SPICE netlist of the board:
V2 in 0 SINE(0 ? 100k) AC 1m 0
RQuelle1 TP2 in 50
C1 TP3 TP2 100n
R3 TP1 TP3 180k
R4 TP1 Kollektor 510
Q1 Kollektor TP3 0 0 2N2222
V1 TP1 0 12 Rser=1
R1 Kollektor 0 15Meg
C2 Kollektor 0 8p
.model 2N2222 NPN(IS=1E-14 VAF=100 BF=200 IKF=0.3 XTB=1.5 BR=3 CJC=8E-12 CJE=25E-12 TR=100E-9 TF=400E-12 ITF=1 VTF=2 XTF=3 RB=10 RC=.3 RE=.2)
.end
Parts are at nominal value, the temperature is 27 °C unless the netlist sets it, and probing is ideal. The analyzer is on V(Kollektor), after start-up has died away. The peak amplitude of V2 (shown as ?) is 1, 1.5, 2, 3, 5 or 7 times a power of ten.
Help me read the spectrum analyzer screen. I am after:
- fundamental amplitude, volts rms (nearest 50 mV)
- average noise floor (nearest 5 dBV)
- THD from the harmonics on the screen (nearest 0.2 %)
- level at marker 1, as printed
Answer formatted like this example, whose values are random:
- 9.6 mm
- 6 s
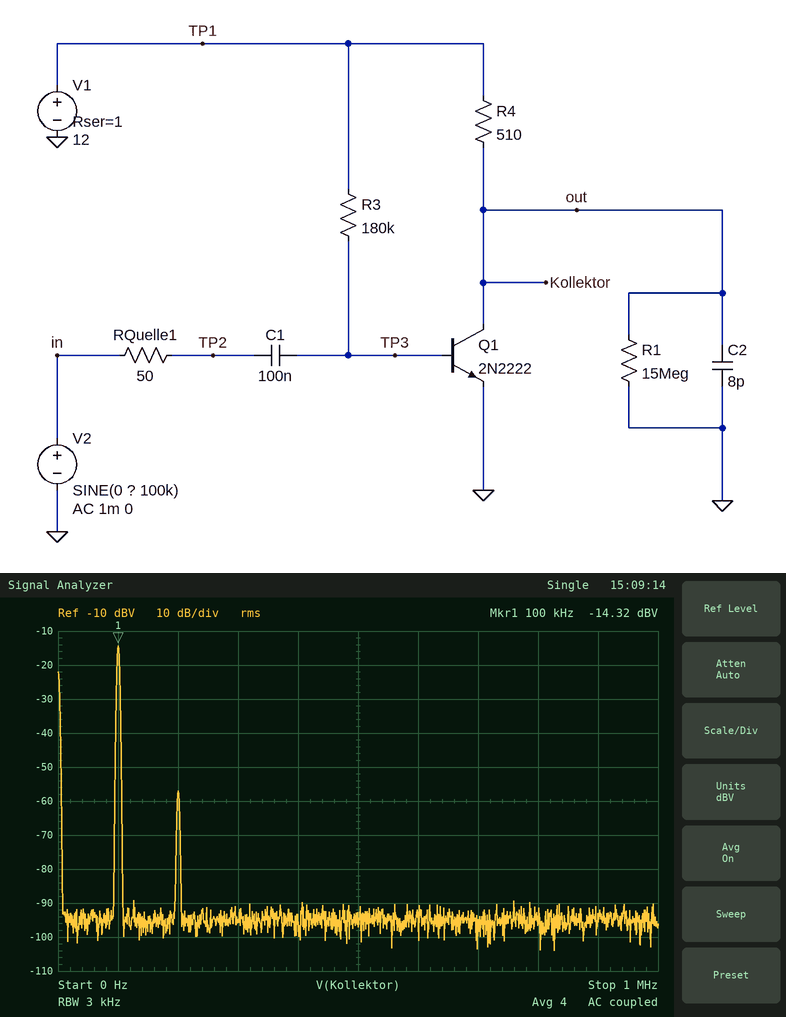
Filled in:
- 200 mV
- -95 dBV
- 0.8 %
- -14.32 dBV
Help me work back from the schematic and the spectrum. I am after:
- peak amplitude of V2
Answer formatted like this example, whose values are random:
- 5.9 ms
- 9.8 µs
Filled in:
- 1.5 mV
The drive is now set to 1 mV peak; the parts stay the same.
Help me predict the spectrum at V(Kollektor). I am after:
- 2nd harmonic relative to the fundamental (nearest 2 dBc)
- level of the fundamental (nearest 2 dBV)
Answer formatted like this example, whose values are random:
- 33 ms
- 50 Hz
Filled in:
- -46 dBc
- -18 dBV
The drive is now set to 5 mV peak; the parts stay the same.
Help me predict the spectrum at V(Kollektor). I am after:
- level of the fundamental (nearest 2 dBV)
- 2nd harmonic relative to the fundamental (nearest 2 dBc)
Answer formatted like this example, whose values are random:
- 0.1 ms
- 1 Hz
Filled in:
- -4 dBV
- -32 dBc
